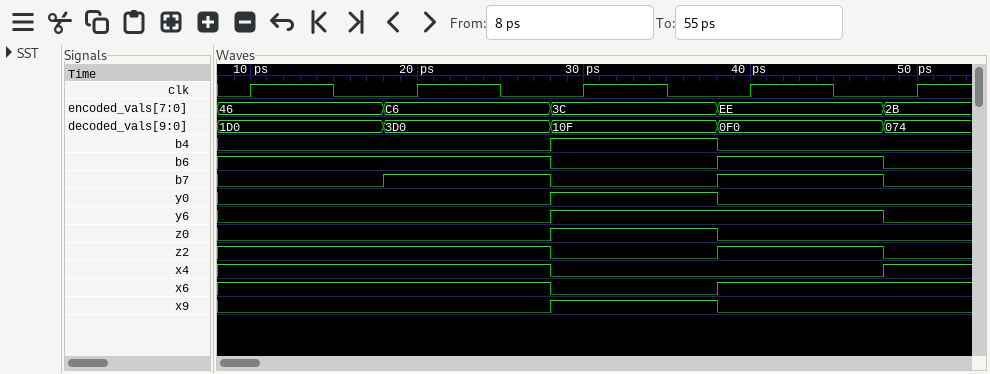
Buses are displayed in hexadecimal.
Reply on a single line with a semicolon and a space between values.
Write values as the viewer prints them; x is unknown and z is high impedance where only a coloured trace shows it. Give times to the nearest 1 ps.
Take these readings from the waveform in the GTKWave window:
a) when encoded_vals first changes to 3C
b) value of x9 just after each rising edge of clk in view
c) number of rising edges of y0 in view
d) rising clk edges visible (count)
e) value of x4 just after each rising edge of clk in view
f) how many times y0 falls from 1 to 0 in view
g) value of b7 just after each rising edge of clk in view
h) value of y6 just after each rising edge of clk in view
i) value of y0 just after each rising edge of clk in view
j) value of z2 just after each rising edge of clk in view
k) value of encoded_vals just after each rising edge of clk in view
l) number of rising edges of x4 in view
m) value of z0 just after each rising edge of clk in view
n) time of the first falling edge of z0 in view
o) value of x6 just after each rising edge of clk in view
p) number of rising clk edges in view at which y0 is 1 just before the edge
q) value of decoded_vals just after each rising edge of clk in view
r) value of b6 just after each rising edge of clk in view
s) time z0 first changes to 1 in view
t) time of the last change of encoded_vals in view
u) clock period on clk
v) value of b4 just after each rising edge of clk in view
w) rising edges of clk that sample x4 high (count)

28 ps; 0 0 1 0 0; 1; 5; 1 1 0 0 1; 1; 0 1 0 1 0; 0 0 1 1 0; 0 0 1 0 0; 1 1 0 1 0; 46, C6, 3C, EE, 2B; 1; 0 0 1 0 0; 38 ps; 1 1 0 1 1; 1; 1D0, 3D0, 10F, 0F0, 074; 1 1 0 1 0; 28 ps; 48 ps; 10 ps; 0 0 1 0 0; 3
